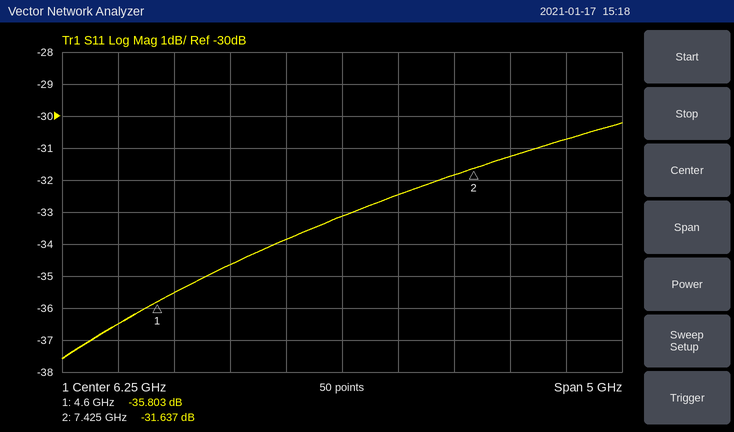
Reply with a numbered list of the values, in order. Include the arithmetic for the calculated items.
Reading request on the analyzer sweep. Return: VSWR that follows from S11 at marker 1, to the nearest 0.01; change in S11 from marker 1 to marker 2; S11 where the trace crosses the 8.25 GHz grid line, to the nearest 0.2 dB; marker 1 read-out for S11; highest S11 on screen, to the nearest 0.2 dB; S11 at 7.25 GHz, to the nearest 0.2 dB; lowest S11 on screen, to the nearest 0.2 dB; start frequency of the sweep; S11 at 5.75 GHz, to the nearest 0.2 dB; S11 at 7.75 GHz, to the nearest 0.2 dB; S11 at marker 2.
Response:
1. (1 + 0.0162)/(1 − 0.0162) ≈ 1.03
2. -31.637 − (-35.803) = 4.166 dB
3. -30.8 dB
4. -35.803 dB
5. -30.2 dB
6. -31.8 dB
7. -37.6 dB
8. 3.75 GHz
9. -33.8 dB
10. -31.2 dB
11. -31.637 dB
